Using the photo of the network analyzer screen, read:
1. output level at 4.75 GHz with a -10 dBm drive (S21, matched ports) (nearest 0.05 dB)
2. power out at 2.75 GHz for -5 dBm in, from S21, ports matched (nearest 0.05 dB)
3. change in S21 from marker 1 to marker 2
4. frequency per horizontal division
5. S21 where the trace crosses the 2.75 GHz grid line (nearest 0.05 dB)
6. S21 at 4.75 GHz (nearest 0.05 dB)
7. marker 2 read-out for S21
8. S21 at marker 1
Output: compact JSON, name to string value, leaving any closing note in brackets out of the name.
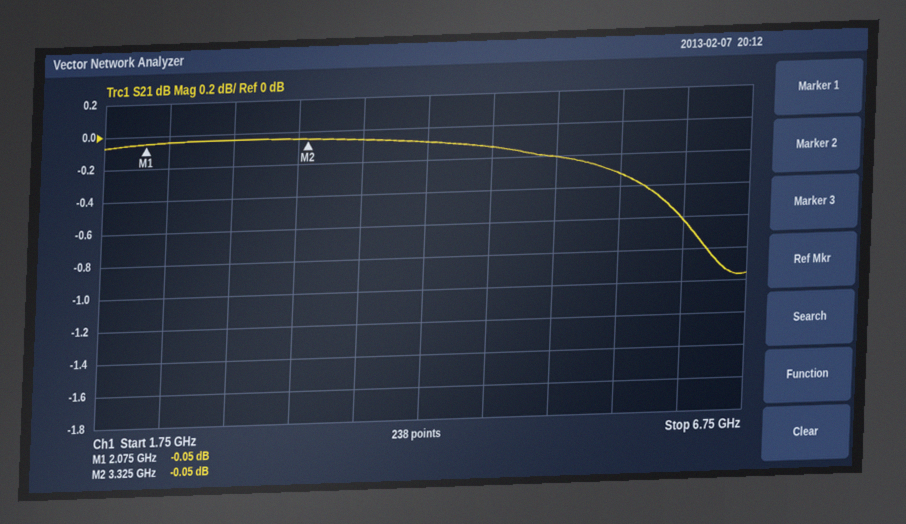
{"output level at 4.75 GHz with a -10 dBm drive (S21, matched ports)": "-10.15 dBm", "power out at 2.75 GHz for -5 dBm in, from S21, ports matched": "-5.05 dBm", "change in S21 from marker 1 to marker 2": "0.00 dB", "frequency per horizontal division": "500 MHz", "S21 where the trace crosses the 2.75 GHz grid line": "-0.05 dB", "S21 at 4.75 GHz": "-0.15 dB", "marker 2 read-out for S21": "-0.05 dB", "S21 at marker 1": "-0.05 dB"}
